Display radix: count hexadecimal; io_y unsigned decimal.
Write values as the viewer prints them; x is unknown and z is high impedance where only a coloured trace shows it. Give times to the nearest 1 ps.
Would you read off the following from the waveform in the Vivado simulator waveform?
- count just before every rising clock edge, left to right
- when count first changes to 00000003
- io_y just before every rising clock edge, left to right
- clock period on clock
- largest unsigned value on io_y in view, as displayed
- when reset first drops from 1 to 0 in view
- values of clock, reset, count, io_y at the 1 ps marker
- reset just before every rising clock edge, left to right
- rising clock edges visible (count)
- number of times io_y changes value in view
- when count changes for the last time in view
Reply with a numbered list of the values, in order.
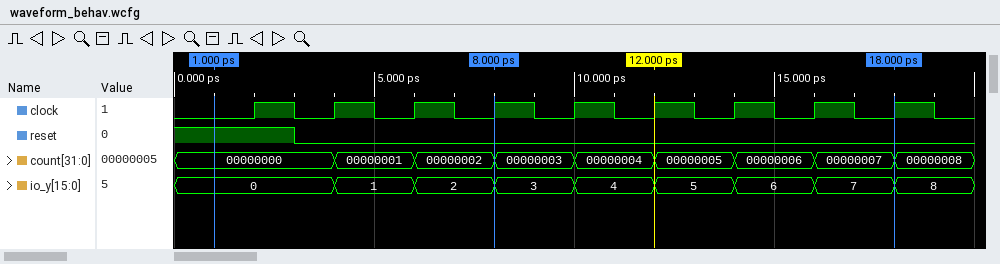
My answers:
1. 00000000, 00000000, 00000001, 00000002, 00000003, 00000004, 00000005, 00000006, 00000007
2. 8 ps
3. 0, 0, 1, 2, 3, 4, 5, 6, 7
4. 2 ps
5. 8
6. 3 ps
7. clock=0, reset=1, count=00000000, io_y=0
8. 1 0 0 0 0 0 0 0 0
9. 9
10. 8
11. 18 ps
